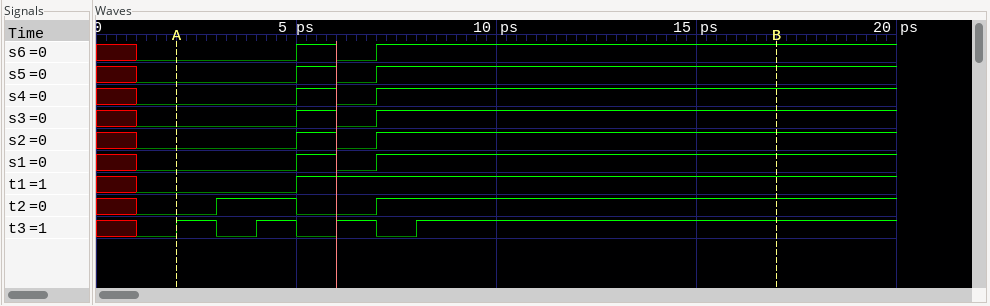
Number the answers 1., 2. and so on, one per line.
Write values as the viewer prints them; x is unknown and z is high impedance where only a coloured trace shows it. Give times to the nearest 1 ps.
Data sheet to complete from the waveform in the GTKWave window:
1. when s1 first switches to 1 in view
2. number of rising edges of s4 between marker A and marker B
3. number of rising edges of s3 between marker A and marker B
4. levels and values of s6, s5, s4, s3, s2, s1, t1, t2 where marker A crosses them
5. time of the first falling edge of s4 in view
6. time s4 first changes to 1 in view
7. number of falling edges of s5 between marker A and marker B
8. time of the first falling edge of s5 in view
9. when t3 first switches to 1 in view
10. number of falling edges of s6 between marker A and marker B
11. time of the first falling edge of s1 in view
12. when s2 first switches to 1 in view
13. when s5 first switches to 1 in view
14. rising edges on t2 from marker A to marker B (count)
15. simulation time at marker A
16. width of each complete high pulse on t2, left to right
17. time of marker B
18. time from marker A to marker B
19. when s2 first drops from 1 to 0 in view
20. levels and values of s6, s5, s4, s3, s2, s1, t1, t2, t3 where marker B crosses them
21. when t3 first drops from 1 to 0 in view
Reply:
1. 5 ps
2. 2
3. 2
4. s6=0, s5=0, s4=0, s3=0, s2=0, s1=0, t1=0, t2=0
5. 6 ps
6. 5 ps
7. 1
8. 6 ps
9. 2 ps
10. 1
11. 6 ps
12. 5 ps
13. 5 ps
14. 2
15. 2 ps
16. 2 ps
17. 17 ps
18. 15 ps
19. 6 ps
20. s6=1, s5=1, s4=1, s3=1, s2=1, s1=1, t1=1, t2=1, t3=1
21. 3 ps
